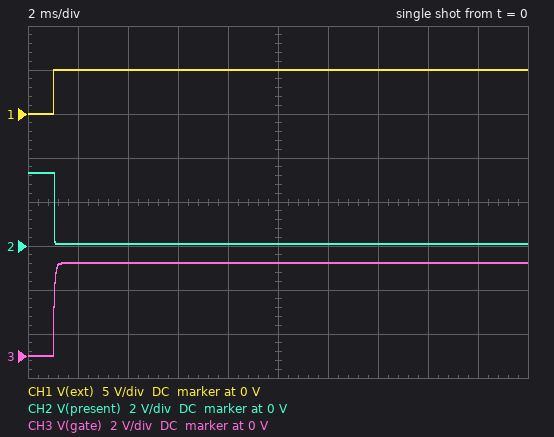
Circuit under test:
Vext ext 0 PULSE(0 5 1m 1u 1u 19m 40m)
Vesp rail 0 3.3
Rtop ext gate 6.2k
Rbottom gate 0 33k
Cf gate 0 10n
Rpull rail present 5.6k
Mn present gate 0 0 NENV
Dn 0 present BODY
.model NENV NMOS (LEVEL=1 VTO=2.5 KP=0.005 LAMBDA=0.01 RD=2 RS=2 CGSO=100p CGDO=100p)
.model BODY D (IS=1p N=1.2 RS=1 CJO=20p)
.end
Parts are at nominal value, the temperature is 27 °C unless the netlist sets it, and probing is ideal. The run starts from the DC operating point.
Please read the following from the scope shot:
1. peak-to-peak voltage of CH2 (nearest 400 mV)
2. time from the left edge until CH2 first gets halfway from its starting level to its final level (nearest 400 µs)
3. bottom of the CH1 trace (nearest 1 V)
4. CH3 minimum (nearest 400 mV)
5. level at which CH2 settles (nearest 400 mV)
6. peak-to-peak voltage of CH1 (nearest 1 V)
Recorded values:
3.2 V
1.2 ms
0 V
0 V
0 V
5 V
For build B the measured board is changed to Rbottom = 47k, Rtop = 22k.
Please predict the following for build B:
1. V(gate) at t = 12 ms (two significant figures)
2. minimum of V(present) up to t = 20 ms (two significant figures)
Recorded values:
3.4 V
140 mV
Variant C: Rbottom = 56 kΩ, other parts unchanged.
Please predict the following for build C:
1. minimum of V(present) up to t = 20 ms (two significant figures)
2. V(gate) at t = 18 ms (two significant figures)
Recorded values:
61 mV
4.5 V
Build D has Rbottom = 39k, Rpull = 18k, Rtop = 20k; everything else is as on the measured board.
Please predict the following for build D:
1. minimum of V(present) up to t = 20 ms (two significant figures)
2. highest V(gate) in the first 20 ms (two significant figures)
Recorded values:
47 mV
3.3 V
